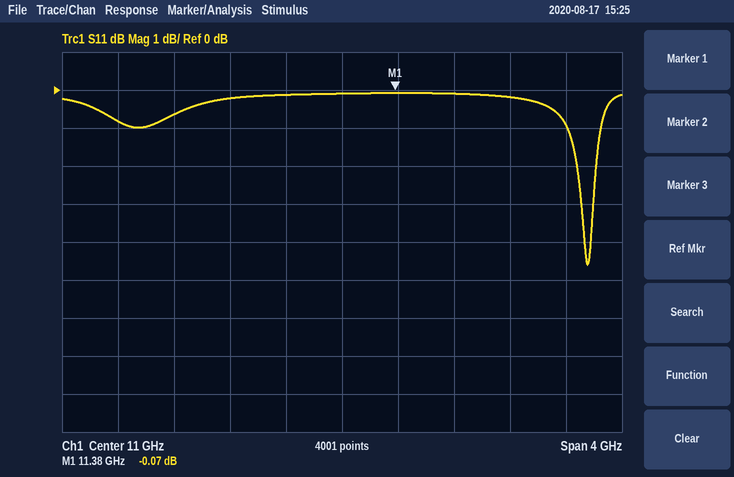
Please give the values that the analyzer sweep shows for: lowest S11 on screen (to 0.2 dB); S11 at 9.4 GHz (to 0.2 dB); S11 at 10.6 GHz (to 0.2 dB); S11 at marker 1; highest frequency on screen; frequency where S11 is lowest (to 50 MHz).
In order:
-4.6 dB
-0.8 dB
-0.2 dB
-0.07 dB
13 GHz
12.75 GHz
